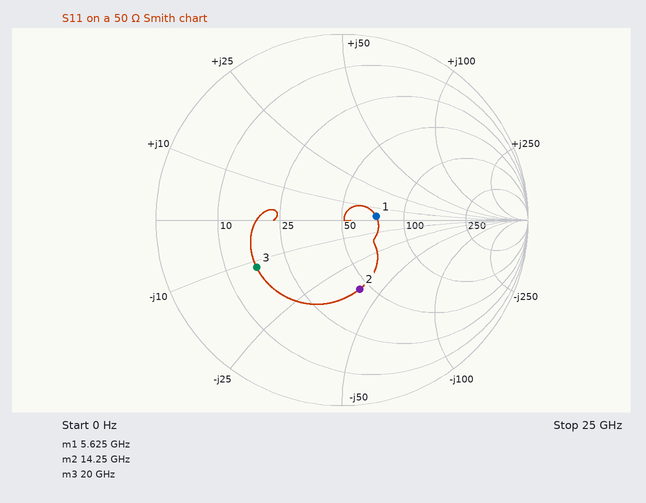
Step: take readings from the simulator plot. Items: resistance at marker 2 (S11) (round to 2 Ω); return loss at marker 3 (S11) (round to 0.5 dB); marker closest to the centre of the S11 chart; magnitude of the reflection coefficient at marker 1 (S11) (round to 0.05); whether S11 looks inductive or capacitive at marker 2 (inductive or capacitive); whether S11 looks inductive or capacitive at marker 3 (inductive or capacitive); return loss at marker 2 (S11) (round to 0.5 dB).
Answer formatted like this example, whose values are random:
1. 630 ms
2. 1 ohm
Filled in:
1. 44 Ω
2. 5.5 dB
3. marker 1
4. 0.20
5. capacitive
6. capacitive
7. 8.5 dB
